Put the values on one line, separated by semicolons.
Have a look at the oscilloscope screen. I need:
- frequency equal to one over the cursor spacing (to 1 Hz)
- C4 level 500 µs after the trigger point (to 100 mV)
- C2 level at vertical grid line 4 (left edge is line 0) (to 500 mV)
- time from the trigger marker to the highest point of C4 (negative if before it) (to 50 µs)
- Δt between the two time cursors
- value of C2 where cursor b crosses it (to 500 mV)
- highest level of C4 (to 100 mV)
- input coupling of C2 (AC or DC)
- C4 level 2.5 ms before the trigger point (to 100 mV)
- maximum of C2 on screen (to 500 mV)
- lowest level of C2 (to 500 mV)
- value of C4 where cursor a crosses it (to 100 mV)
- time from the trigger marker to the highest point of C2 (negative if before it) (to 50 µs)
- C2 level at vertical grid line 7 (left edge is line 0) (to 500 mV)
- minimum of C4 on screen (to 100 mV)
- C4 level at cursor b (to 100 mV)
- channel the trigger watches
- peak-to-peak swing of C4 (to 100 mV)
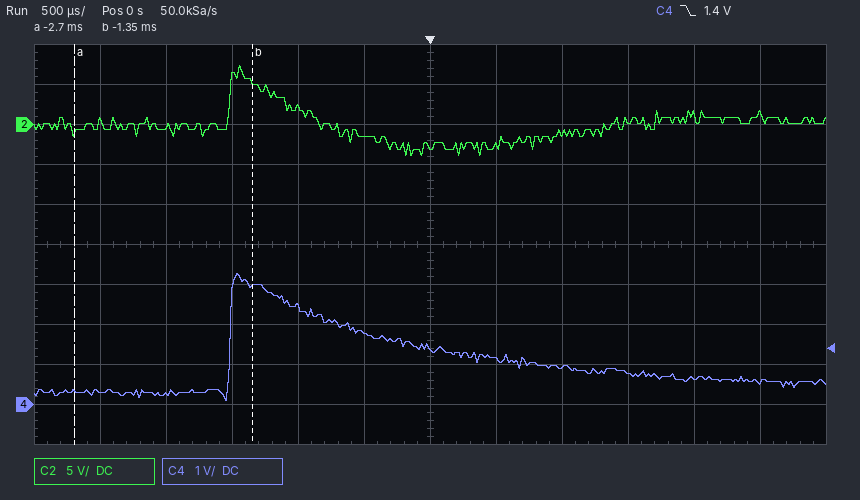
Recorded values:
741 Hz; 1.1 V; 2.0 V; -1.45 ms; 1.35 ms; 5.5 V; 3.3 V; DC; 300 mV; 7.5 V; -4.0 V; 300 mV; -1.45 ms; -2.5 V; 100 mV; 3.0 V; C4; 3.2 V
